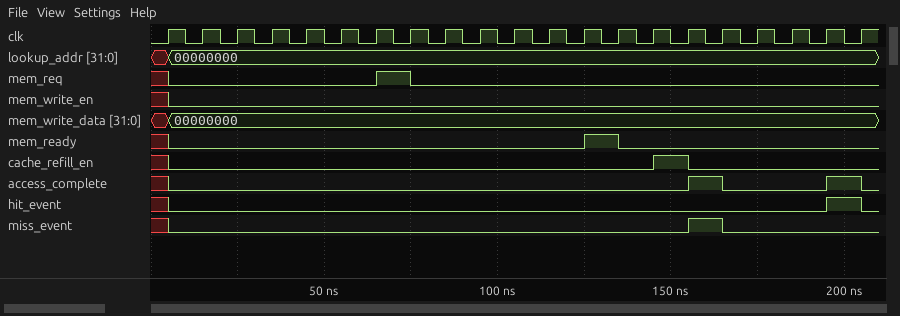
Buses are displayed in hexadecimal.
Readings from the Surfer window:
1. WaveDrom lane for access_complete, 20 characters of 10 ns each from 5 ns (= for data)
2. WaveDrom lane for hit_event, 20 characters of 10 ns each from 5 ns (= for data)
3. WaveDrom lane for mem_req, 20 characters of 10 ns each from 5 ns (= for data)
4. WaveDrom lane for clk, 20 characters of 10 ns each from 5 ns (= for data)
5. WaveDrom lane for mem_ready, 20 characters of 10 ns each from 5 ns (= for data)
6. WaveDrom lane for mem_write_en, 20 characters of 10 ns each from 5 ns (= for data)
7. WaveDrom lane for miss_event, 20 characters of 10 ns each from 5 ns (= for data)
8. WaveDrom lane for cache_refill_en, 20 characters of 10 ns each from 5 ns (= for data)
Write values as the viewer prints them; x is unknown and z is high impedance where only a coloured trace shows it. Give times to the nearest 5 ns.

{name: 'access_complete', wave: '0..............10..1'}
{name: 'hit_event', wave: '0..................1'}
{name: 'mem_req', wave: '0.....10............'}
{name: 'clk', wave: 'p...................'}
{name: 'mem_ready', wave: '0...........10......'}
{name: 'mem_write_en', wave: '0...................'}
{name: 'miss_event', wave: '0..............10...'}
{name: 'cache_refill_en', wave: '0.............10....'}
